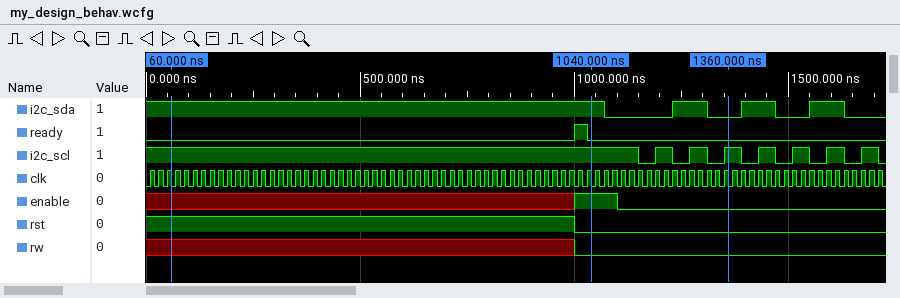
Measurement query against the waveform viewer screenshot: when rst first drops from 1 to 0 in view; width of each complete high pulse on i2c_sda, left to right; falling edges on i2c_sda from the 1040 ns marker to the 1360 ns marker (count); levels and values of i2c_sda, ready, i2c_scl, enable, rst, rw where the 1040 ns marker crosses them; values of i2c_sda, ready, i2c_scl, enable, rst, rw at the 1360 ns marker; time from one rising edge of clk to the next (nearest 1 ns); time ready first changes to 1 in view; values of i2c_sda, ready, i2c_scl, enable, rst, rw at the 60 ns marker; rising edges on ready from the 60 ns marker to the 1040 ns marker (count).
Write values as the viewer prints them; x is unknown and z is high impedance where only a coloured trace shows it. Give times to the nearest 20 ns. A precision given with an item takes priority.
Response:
1000 ns
80 ns, 80 ns, 80 ns
2
i2c_sda=1, ready=0, i2c_scl=1, enable=1, rst=0, rw=0
i2c_sda=0, ready=0, i2c_scl=1, enable=0, rst=0, rw=0
20 ns
1000 ns
i2c_sda=1, ready=0, i2c_scl=1, enable=x, rst=1, rw=x
1
